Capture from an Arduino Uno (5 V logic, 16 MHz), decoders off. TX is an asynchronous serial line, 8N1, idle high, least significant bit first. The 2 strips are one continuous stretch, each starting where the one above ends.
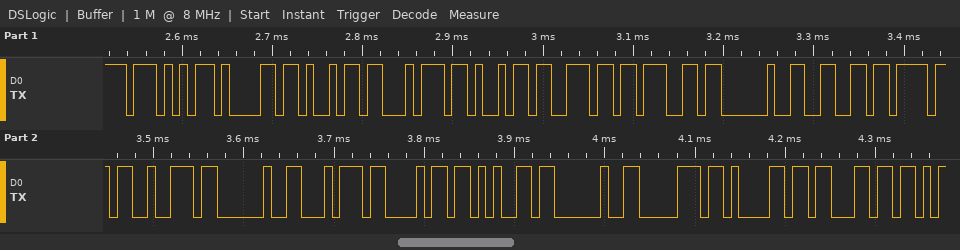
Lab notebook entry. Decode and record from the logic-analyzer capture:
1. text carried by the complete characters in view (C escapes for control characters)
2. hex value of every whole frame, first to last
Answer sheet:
"Waiting for the pac"
57 61 69 74 69 6E 67 20 66 6F 72 20 74 68 65 20 70 61 63
